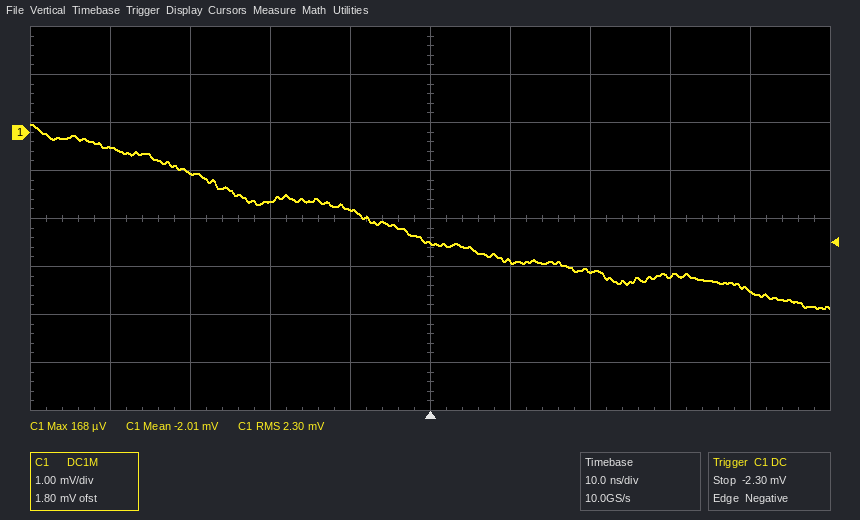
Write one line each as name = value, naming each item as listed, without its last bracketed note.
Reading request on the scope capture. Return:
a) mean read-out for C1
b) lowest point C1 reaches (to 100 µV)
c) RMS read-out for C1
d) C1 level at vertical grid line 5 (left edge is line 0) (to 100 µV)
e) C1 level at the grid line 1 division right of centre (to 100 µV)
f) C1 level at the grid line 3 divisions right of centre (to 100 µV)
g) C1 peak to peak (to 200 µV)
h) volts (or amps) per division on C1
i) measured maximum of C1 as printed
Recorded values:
mean read-out for C1 = -2.01 mV
lowest point C1 reaches = -3.7 mV
RMS read-out for C1 = 2.30 mV
C1 level at vertical grid line 5 (left edge is line 0) = -2.3 mV
C1 level at the grid line 1 division right of centre = -2.7 mV
C1 level at the grid line 3 divisions right of centre = -3.0 mV
C1 peak to peak = 3.8 mV
volts (or amps) per division on C1 = 1 mV
measured maximum of C1 as printed = 168 µV
